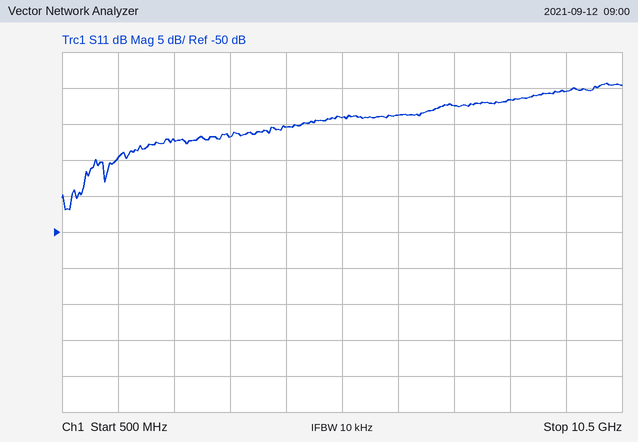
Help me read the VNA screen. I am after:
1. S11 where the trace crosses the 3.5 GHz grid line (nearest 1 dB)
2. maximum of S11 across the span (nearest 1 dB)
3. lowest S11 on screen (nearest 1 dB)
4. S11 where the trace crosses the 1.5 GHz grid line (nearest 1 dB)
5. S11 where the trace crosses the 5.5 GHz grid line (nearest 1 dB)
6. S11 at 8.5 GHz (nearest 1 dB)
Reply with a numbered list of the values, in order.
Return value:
1. -37 dB
2. -29 dB
3. -47 dB
4. -40 dB
5. -34 dB
6. -32 dB
